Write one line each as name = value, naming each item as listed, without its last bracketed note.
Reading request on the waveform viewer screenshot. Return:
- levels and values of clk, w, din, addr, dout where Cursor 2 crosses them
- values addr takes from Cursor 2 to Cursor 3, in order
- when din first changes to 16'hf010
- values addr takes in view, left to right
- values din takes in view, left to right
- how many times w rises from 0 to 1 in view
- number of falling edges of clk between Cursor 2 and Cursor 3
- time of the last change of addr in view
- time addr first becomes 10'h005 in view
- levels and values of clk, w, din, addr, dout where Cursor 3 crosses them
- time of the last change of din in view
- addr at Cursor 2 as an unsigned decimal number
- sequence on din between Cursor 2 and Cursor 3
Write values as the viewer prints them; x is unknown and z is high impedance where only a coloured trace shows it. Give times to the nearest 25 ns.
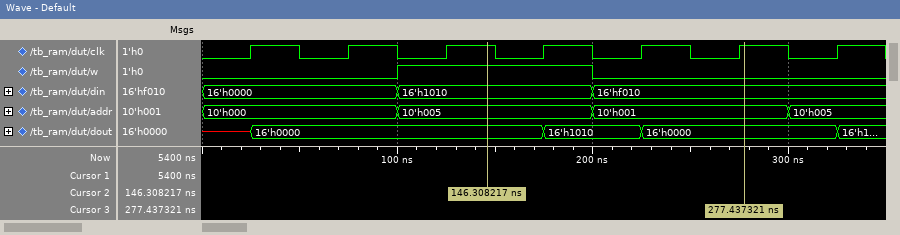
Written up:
levels and values of clk, w, din, addr, dout where Cursor 2 crosses them = clk=1, w=1, din=16'h1010, addr=10'h005, dout=16'h0000
values addr takes from Cursor 2 to Cursor 3, in order = 10'h005, 10'h001
when din first changes to 16'hf010 = 200 ns
values addr takes in view, left to right = 10'h000, 10'h005, 10'h001, 10'h005
values din takes in view, left to right = 16'h0000, 16'h1010, 16'hf010
how many times w rises from 0 to 1 in view = 1
number of falling edges of clk between Cursor 2 and Cursor 3 = 3
time of the last change of addr in view = 300 ns
time addr first becomes 10'h005 in view = 100 ns
levels and values of clk, w, din, addr, dout where Cursor 3 crosses them = clk=1, w=0, din=16'hf010, addr=10'h001, dout=16'h0000
time of the last change of din in view = 200 ns
addr at Cursor 2 as an unsigned decimal number = 5
sequence on din between Cursor 2 and Cursor 3 = 16'h1010, 16'hf010
